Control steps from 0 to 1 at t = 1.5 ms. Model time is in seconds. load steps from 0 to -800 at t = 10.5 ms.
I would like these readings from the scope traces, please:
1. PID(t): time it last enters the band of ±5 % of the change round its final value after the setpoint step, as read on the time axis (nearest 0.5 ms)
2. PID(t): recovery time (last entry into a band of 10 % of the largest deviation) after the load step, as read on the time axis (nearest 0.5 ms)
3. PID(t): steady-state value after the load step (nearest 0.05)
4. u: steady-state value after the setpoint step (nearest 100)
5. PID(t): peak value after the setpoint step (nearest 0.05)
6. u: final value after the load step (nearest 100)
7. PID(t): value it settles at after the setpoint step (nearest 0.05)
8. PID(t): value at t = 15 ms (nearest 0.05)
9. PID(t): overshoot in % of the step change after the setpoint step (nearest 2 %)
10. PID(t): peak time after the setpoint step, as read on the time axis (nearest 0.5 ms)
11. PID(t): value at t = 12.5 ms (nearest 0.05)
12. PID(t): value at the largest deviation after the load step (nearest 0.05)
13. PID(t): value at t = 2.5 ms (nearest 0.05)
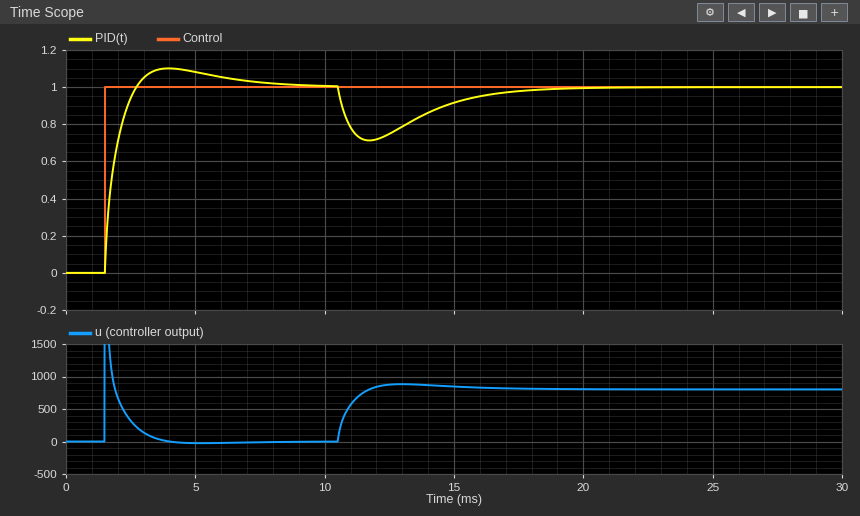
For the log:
6.0 ms
17.0 ms
1.00
0
1.10
800
1.00
0.90
10 %
4.0 ms
0.75
0.70
0.95
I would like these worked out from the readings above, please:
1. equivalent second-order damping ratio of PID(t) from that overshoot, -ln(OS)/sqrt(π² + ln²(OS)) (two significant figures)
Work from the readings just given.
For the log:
0.59
